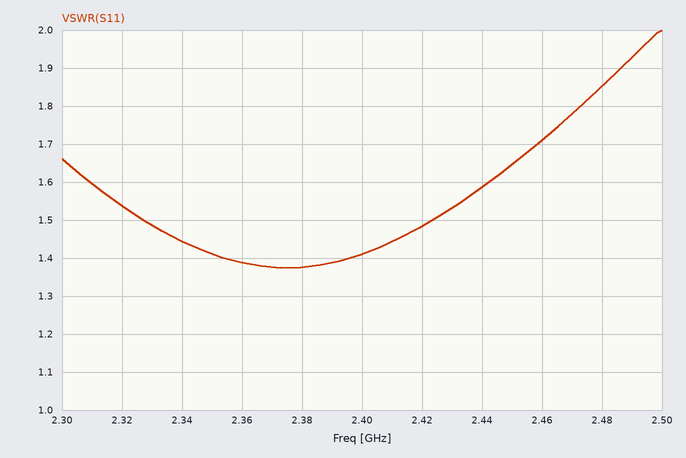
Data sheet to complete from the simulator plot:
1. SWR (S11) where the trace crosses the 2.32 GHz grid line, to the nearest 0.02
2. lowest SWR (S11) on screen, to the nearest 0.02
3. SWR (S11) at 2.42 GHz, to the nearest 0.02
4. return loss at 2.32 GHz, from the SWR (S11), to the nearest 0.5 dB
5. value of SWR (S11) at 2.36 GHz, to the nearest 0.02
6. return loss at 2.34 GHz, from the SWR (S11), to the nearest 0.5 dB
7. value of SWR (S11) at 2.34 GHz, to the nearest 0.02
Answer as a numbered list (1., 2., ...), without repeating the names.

1. 1.54
2. 1.38
3. 1.48
4. 13.5 dB
5. 1.38
6. 15.0 dB
7. 1.44
